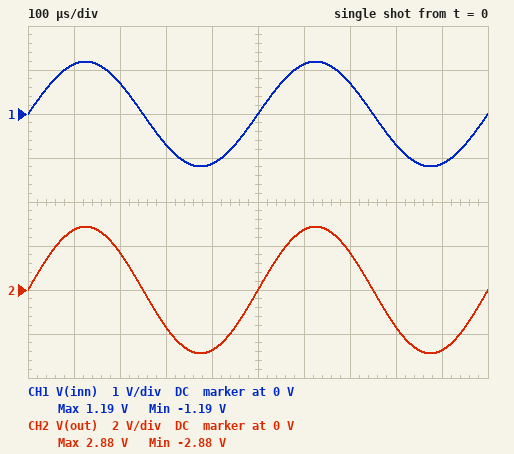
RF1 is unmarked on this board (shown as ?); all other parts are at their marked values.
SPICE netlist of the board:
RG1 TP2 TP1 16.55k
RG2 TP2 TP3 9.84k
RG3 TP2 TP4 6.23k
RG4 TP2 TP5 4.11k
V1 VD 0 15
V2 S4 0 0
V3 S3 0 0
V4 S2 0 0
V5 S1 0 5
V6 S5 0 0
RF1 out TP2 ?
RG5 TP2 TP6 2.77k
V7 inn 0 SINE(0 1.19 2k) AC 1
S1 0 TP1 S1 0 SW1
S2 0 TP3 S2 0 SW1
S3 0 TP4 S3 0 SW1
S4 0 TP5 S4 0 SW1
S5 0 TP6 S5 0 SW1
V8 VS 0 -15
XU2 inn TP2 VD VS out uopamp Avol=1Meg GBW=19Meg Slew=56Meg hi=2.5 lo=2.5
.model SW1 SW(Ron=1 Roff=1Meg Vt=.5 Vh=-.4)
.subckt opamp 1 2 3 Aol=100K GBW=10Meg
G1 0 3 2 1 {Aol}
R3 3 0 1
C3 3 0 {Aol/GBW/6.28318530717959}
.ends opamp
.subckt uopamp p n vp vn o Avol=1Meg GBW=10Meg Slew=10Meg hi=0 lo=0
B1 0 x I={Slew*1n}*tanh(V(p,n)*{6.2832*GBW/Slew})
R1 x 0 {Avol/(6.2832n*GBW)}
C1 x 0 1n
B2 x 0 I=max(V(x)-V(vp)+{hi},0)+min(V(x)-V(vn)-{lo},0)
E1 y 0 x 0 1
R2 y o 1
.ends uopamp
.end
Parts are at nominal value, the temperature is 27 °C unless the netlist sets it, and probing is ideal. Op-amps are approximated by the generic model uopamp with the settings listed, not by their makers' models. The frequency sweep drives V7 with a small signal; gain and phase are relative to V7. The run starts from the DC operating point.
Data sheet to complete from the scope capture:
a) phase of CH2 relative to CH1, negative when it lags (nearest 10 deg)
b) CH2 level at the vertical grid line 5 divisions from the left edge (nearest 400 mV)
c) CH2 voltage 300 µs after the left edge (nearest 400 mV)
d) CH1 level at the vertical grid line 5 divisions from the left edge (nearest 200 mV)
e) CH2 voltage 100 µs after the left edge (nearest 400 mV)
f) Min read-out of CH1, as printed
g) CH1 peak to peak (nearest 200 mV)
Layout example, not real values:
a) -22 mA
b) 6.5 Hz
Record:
a) 0 deg
b) 0 V
c) -1.6 V
d) 0 V
e) 2.8 V
f) -1.19 V
g) 2.4 V
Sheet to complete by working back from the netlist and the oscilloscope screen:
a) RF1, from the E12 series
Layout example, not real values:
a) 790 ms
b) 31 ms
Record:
a) 22 kΩ
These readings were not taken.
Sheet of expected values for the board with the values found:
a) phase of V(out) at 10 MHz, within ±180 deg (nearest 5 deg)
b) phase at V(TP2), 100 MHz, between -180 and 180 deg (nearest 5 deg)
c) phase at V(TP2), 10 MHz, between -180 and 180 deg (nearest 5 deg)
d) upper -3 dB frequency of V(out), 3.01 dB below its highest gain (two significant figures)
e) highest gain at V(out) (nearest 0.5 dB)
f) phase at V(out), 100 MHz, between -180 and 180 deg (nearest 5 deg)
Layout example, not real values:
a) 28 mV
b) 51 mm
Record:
a) -30 deg
b) -80 deg
c) -30 deg
d) 17 MHz
e) 1.0 dB
f) -80 deg
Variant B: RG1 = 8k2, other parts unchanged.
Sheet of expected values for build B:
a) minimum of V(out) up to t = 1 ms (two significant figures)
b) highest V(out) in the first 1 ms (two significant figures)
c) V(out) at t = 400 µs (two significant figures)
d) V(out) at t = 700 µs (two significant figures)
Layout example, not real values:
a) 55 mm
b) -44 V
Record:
a) -4.5 V
b) 4.5 V
c) -4.3 V
d) 2.6 V
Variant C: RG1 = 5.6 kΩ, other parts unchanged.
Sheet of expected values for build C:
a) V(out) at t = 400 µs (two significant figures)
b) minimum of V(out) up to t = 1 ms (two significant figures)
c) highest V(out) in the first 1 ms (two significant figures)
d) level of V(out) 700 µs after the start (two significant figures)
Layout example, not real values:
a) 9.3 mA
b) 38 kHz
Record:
a) -5.7 V
b) -6.0 V
c) 6.0 V
d) 3.5 V
